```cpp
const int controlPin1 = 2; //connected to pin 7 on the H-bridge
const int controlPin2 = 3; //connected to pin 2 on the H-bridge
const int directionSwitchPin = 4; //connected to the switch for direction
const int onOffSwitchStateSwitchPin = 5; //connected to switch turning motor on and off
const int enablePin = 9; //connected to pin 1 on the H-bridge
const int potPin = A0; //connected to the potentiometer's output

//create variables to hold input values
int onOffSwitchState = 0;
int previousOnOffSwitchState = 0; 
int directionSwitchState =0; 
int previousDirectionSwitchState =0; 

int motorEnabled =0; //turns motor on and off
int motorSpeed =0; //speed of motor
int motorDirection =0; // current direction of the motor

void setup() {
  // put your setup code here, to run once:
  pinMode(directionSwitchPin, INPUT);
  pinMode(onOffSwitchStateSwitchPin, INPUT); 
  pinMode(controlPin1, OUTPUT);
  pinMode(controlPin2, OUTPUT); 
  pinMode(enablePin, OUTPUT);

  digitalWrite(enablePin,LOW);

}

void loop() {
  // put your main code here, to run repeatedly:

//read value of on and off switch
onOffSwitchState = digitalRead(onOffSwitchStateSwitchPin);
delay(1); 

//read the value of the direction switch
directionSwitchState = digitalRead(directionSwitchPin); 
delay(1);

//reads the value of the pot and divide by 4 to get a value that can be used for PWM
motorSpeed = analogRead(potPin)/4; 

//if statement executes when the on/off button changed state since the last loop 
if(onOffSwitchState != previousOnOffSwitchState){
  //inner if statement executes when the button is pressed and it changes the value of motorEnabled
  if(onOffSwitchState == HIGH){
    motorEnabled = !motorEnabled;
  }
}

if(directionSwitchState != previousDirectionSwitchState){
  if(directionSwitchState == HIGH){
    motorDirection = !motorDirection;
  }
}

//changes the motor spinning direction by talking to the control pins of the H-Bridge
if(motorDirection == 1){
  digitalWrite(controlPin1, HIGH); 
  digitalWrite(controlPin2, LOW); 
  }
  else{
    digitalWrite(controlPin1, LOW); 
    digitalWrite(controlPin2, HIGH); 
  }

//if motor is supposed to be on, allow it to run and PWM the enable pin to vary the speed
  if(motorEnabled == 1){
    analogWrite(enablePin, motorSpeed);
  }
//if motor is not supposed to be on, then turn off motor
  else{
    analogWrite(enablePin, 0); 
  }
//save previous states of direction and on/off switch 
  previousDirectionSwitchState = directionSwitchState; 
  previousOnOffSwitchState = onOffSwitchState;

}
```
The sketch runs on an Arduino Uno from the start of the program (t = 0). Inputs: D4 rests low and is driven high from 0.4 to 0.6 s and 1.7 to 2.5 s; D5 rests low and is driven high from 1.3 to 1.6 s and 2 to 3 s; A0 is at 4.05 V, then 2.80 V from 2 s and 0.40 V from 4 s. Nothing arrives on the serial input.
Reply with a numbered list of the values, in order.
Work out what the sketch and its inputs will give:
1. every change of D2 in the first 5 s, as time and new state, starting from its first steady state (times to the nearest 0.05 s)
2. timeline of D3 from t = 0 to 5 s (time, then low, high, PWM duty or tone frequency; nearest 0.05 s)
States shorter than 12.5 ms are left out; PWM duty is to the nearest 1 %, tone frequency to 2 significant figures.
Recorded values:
1. 0 s low; 0.4 s high; 1.7 s low
2. 0 s high; 0.4 s low; 1.7 s high
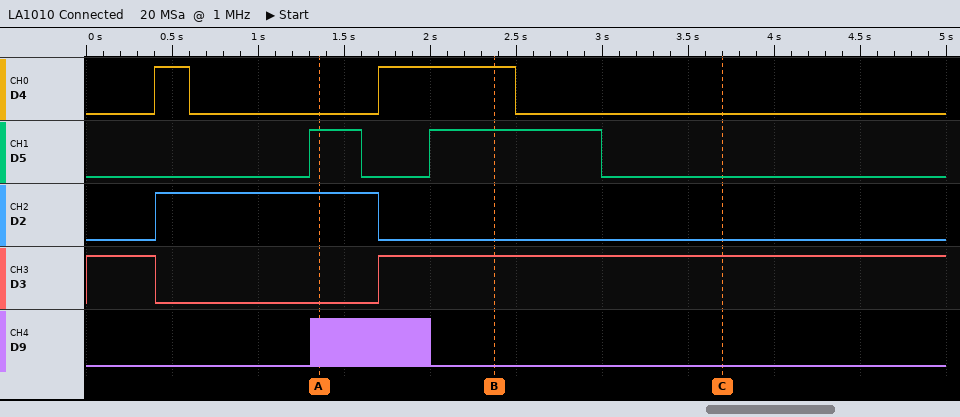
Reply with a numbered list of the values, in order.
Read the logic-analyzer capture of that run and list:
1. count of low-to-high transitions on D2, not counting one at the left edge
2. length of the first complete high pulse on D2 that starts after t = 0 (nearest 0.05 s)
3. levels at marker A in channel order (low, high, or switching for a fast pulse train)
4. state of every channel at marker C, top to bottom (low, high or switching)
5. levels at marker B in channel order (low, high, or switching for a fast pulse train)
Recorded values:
1. 1
2. 1.30 s
3. D4 low, D5 high, D2 high, D3 low, D9 switching
4. D4 low, D5 low, D2 low, D3 high, D9 low
5. D4 high, D5 high, D2 low, D3 high, D9 low
